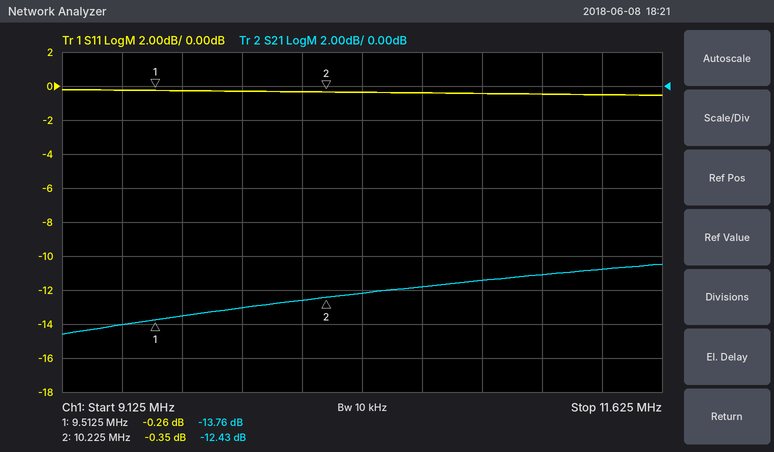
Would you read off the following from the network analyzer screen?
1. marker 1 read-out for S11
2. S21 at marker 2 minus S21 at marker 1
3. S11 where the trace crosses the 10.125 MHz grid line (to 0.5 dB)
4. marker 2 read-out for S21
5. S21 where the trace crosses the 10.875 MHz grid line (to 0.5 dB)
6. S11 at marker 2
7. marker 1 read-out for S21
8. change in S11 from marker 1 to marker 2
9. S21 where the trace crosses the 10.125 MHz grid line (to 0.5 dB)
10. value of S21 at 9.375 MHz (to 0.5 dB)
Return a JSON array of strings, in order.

["-0.26 dB", "1.33 dB", "-0.5 dB", "-12.43 dB", "-11.5 dB", "-0.35 dB", "-13.76 dB", "-0.09 dB", "-12.5 dB", "-14.0 dB"]
